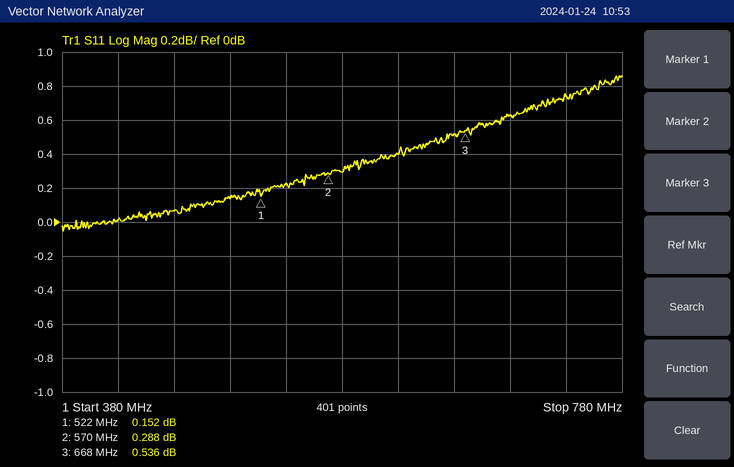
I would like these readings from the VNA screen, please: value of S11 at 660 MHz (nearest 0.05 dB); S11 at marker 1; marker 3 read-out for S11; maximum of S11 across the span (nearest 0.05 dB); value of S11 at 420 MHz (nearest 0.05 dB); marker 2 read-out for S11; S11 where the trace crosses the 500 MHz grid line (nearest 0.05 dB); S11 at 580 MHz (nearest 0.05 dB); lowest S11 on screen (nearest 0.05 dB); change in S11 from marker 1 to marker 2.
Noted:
0.50 dB
0.152 dB
0.536 dB
0.85 dB
0.00 dB
0.288 dB
0.15 dB
0.30 dB
-0.05 dB
0.136 dB
